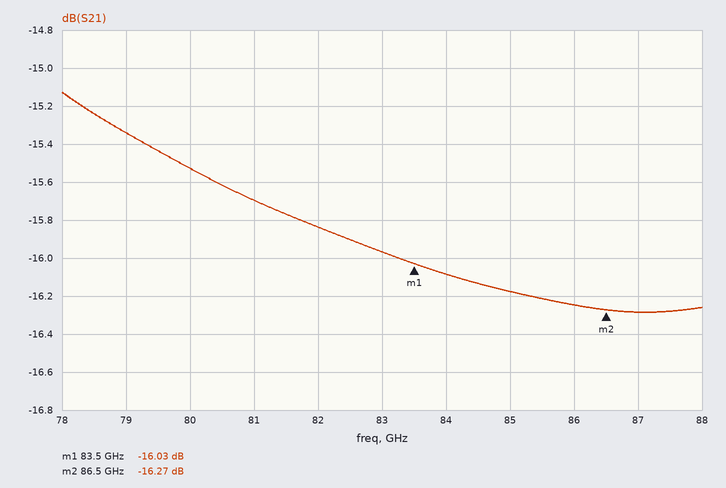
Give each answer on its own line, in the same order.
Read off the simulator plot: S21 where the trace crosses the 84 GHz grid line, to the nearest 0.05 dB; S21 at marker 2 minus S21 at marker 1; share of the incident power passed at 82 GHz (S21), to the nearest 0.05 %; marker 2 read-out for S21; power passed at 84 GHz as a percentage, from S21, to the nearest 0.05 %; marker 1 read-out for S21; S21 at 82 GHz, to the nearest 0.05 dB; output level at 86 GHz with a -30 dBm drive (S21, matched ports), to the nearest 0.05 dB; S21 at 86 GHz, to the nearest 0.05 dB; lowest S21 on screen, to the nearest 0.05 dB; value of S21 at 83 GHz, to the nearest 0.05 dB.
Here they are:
-16.10 dB
-0.24 dB
2.60 %
-16.27 dB
2.45 %
-16.03 dB
-15.85 dB
-46.25 dBm
-16.25 dB
-16.30 dB
-15.95 dB
